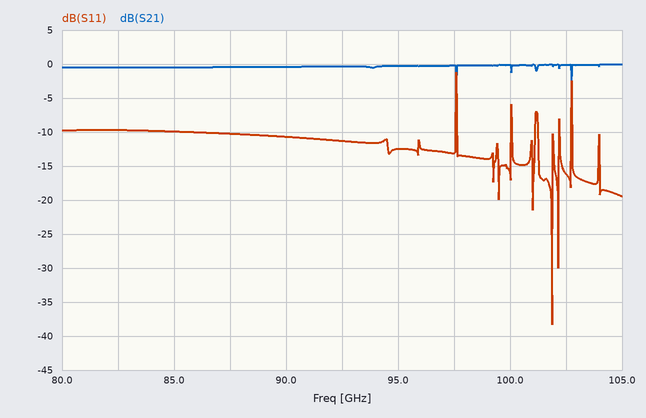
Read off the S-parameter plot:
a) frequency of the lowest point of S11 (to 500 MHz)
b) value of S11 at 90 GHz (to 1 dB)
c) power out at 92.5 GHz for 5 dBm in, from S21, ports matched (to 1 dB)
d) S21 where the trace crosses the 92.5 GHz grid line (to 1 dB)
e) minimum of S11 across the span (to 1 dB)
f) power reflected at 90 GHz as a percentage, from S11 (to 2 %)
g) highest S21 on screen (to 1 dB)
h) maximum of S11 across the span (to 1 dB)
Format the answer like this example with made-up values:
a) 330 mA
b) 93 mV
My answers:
a) 102.0 GHz
b) -11 dB
c) 5 dBm
d) 0 dB
e) -38 dB
f) 8 %
g) 0 dB
h) -1 dB
